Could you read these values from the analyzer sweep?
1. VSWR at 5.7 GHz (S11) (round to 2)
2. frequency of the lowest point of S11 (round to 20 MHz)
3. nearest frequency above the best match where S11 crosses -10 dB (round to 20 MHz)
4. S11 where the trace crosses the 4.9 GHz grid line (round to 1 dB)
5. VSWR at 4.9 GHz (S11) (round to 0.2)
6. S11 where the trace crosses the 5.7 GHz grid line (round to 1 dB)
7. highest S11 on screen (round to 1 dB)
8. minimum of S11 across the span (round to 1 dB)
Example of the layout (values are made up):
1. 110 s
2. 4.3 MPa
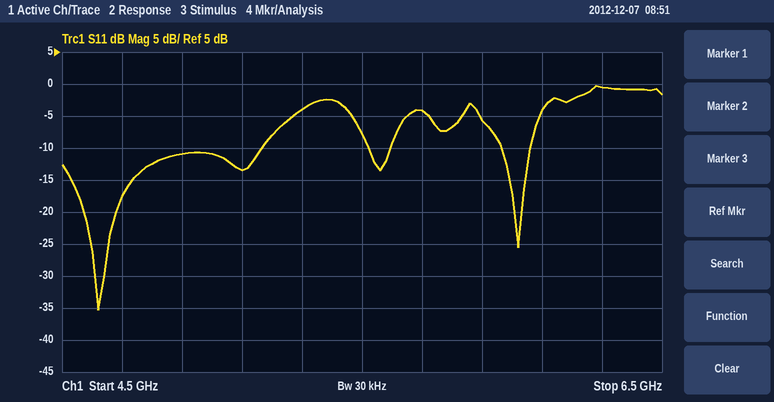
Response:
1. 4
2. 4.62 GHz
3. 5.16 GHz
4. -11 dB
5. 1.8
6. -4 dB
7. 0 dB
8. -35 dB
